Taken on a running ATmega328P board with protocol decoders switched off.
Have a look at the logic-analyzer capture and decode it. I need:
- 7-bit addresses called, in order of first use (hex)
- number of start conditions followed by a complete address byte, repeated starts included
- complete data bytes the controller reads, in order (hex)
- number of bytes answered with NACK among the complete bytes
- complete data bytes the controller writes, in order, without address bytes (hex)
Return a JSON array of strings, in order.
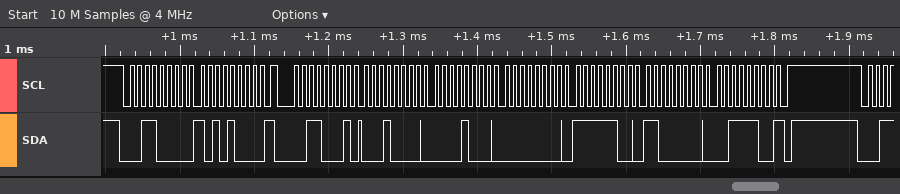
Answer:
["0x18", "2", "10 08 00 FC C0 3C", "1", "A8"]
